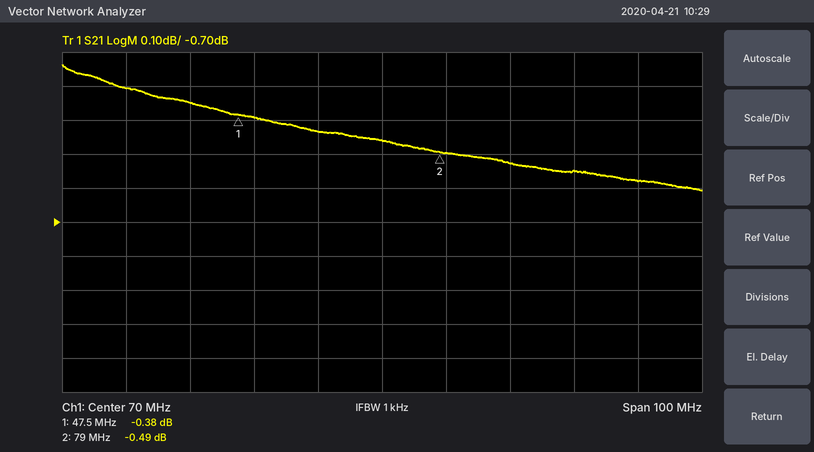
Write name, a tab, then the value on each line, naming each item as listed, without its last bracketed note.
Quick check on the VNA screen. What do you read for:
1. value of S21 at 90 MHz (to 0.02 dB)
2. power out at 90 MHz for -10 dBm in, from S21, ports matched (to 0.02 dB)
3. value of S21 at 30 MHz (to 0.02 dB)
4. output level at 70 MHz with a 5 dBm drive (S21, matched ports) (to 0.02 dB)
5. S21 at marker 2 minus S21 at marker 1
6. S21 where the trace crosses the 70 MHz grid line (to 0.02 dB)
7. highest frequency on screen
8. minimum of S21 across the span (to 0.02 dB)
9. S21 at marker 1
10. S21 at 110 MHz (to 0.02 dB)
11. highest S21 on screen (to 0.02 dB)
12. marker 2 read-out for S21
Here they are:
value of S21 at 90 MHz	-0.52 dB
power out at 90 MHz for -10 dBm in, from S21, ports matched	-10.52 dBm
value of S21 at 30 MHz	-0.30 dB
output level at 70 MHz with a 5 dBm drive (S21, matched ports)	4.54 dBm
S21 at marker 2 minus S21 at marker 1	-0.11 dB
S21 where the trace crosses the 70 MHz grid line	-0.46 dB
highest frequency on screen	120 MHz
minimum of S21 across the span	-0.60 dB
S21 at marker 1	-0.38 dB
S21 at 110 MHz	-0.58 dB
highest S21 on screen	-0.24 dB
marker 2 read-out for S21	-0.49 dB
